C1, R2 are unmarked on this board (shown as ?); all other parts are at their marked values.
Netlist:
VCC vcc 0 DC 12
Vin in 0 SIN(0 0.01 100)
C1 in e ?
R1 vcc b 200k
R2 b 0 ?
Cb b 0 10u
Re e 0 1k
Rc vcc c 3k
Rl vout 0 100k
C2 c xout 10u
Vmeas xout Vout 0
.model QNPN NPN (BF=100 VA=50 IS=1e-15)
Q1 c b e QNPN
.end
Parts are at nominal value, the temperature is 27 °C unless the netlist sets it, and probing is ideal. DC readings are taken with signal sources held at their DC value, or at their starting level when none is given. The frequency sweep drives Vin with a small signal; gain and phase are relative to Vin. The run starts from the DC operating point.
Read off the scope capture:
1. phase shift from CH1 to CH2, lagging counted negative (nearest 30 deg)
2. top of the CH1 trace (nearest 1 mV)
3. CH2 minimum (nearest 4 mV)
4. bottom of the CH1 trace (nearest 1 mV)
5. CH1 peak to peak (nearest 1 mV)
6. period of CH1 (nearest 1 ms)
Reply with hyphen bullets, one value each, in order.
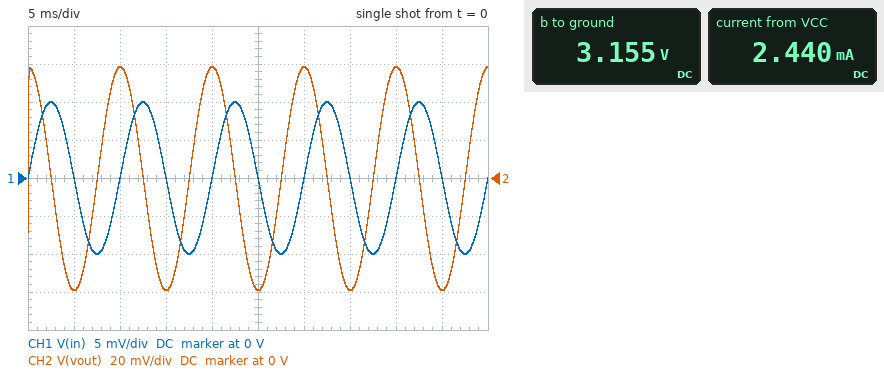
- 90 deg
- 10 mV
- -60 mV
- -10 mV
- 20 mV
- 10 ms
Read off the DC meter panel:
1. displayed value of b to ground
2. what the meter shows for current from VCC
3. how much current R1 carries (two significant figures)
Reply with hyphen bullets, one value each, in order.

- 3.155 V
- 2.440 mA
- 44 µA
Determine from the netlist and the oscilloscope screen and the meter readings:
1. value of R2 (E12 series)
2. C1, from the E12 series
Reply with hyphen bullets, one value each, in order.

- 150 kΩ
- 3.3 µF
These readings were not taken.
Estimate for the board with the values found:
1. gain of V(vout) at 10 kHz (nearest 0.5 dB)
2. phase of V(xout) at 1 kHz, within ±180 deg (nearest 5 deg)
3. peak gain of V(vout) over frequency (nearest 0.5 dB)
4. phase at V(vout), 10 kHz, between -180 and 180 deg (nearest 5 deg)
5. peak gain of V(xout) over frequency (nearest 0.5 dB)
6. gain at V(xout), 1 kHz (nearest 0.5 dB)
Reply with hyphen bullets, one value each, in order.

- 47.0 dB
- 75 deg
- 47.5 dB
- 20 deg
- 47.5 dB
- 35.0 dB
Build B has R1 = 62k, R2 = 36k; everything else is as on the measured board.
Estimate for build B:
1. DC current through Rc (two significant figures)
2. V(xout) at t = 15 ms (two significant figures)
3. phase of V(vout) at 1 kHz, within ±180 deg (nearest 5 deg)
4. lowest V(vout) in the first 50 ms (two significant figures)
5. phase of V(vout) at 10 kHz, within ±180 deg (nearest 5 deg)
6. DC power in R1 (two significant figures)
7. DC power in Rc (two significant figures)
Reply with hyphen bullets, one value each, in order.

- 2.9 mA
- -43 mV
- 80 deg
- -44 mV
- 25 deg
- 1.1 mW
- 26 mW
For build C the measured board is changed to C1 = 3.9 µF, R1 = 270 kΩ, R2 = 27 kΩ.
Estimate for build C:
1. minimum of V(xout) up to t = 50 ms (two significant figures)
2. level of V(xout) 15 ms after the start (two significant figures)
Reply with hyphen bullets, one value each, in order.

- -65 mV
- -64 mV
